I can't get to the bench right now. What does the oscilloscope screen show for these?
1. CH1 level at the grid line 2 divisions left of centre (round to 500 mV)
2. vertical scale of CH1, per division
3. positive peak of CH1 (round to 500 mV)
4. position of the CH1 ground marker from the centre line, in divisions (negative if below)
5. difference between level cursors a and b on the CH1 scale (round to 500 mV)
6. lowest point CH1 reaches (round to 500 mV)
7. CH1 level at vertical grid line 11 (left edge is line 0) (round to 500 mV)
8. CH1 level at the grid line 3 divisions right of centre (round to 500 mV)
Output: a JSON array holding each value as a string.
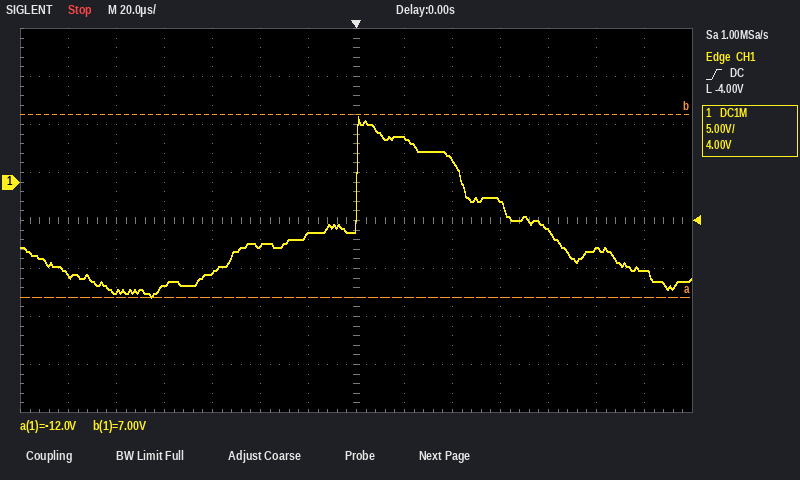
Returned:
["-6.5 V", "5 V", "7.0 V", "+0.8 div", "19.0 V", "-12.0 V", "-5.0 V", "-2.0 V"]
